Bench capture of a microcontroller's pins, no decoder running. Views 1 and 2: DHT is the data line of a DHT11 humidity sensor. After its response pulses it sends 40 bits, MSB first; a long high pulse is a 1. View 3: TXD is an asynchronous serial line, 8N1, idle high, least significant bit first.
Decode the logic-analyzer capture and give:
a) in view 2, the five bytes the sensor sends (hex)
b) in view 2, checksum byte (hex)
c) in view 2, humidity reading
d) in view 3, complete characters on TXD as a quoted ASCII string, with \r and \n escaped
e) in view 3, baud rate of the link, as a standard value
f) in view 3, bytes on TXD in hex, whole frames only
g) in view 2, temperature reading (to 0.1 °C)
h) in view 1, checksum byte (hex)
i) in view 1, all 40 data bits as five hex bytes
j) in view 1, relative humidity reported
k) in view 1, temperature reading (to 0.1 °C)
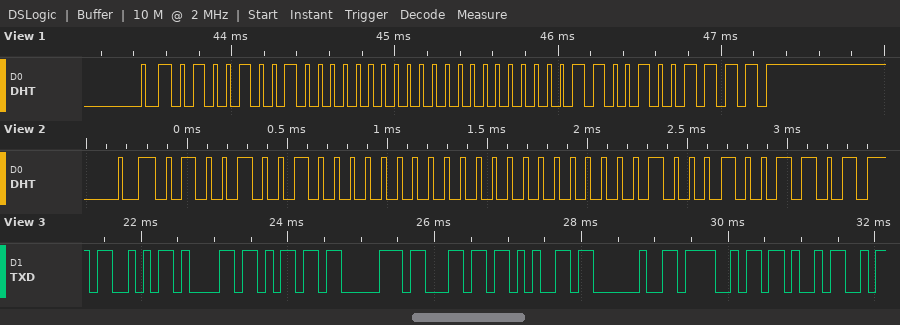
49 00 00 04 4D
0x4D
73 %
"Sample OK"
9600 baud
53 61 6D 70 6C 65 20 4F 4B
0.4 °C
0x4F
49 00 00 06 4F
73 %
0.6 °C
